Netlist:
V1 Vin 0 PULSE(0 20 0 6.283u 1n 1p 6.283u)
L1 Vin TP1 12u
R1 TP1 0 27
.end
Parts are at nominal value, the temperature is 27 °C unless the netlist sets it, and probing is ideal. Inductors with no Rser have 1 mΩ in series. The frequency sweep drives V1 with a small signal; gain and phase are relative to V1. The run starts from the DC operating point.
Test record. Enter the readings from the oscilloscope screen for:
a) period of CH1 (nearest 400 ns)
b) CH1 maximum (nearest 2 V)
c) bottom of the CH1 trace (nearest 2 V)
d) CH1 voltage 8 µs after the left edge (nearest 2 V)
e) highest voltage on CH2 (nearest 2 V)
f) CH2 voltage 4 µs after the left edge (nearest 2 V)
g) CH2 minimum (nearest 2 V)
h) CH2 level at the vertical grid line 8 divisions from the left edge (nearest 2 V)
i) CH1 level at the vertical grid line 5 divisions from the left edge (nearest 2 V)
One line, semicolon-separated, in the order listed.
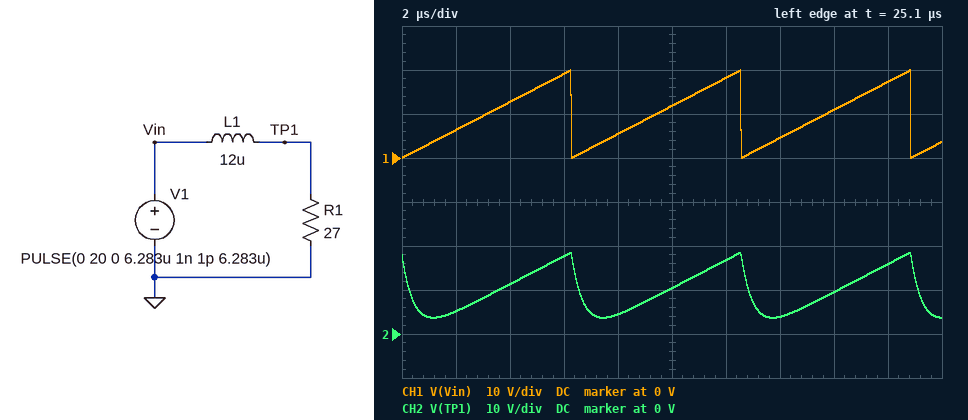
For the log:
6.4 µs; 20 V; 0 V; 6 V; 18 V; 12 V; 4 V; 10 V; 12 V
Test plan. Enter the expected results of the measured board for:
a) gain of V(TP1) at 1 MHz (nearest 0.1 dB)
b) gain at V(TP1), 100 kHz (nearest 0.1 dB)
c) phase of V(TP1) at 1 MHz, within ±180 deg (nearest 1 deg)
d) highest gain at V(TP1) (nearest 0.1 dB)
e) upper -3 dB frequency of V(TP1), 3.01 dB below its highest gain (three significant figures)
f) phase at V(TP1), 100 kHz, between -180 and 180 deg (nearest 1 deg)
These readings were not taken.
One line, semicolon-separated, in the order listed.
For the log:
-9.4 dB; -0.3 dB; -70 deg; 0 dB; 358 kHz; -16 deg
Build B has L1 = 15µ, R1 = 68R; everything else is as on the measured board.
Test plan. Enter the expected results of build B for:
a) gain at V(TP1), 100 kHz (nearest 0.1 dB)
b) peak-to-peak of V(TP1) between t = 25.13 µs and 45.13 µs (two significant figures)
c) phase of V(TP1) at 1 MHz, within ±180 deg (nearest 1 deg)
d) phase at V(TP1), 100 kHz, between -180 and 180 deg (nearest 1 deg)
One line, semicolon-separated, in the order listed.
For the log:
-0.1 dB; 17 V; -54 deg; -8 deg
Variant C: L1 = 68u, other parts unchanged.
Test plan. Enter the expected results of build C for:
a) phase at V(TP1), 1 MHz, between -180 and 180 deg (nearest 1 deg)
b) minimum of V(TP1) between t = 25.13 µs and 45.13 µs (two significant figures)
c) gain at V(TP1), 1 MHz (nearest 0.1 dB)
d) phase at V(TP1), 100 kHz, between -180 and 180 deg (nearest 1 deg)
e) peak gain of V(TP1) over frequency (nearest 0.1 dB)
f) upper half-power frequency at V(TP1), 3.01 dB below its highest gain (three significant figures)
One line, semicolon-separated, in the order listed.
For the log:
-86 deg; 8.0 V; -24.0 dB; -58 deg; 0 dB; 63.2 kHz
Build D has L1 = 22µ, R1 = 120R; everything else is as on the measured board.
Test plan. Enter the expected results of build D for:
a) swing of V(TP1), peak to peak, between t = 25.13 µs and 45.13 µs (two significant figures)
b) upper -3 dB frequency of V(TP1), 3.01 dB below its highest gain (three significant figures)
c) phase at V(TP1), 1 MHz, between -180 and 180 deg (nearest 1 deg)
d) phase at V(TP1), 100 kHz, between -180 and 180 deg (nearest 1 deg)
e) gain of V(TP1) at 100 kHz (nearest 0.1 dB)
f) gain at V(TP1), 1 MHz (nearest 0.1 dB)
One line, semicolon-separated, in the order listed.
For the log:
17 V; 868 kHz; -49 deg; -7 deg; -0.1 dB; -3.7 dB
